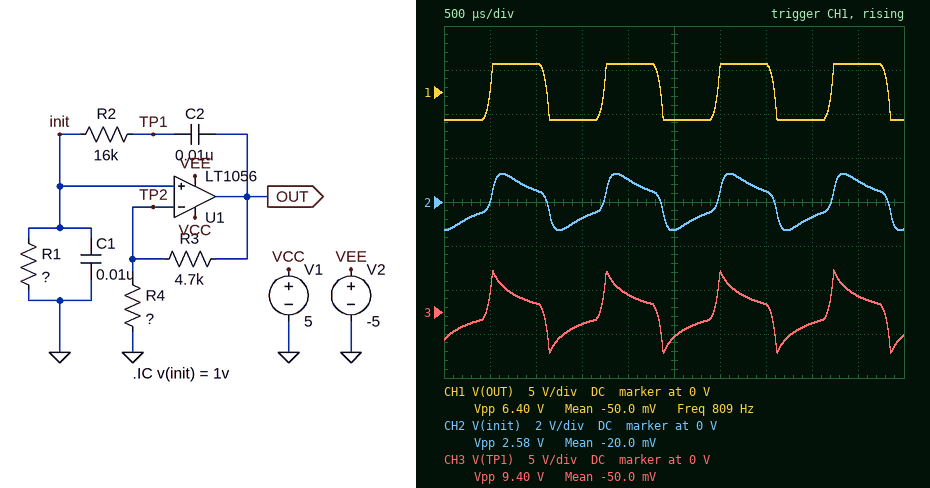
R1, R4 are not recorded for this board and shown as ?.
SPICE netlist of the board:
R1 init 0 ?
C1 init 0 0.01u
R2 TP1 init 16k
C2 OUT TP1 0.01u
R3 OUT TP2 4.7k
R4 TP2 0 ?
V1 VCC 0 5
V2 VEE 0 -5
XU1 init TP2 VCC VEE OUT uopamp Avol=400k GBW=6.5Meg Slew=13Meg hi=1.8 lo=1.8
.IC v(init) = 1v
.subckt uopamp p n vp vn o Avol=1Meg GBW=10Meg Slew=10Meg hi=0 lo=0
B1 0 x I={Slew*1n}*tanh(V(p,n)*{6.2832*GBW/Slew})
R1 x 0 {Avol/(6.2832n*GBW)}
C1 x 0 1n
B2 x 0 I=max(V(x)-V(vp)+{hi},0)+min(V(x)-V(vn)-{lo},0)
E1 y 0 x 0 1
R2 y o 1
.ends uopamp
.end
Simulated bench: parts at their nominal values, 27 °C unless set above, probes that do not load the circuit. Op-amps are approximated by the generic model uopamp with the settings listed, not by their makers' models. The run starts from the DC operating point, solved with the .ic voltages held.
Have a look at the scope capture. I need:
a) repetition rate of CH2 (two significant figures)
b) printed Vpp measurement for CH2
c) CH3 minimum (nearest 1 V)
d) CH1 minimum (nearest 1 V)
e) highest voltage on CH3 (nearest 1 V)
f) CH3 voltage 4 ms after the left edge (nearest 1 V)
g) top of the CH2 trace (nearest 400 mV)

810 Hz
2.58 V
-5 V
-3 V
5 V
-1 V
1.2 V
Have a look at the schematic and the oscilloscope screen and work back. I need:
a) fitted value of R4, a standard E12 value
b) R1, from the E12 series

820 Ω
12 kΩ
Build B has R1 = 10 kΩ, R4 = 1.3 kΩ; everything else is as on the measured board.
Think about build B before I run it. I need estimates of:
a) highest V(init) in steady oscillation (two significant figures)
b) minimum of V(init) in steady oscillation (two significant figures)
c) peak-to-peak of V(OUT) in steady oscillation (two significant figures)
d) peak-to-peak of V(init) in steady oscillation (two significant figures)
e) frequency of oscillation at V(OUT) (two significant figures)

1.1 V
-1.1 V
6.4 V
2.1 V
1.1 kHz
